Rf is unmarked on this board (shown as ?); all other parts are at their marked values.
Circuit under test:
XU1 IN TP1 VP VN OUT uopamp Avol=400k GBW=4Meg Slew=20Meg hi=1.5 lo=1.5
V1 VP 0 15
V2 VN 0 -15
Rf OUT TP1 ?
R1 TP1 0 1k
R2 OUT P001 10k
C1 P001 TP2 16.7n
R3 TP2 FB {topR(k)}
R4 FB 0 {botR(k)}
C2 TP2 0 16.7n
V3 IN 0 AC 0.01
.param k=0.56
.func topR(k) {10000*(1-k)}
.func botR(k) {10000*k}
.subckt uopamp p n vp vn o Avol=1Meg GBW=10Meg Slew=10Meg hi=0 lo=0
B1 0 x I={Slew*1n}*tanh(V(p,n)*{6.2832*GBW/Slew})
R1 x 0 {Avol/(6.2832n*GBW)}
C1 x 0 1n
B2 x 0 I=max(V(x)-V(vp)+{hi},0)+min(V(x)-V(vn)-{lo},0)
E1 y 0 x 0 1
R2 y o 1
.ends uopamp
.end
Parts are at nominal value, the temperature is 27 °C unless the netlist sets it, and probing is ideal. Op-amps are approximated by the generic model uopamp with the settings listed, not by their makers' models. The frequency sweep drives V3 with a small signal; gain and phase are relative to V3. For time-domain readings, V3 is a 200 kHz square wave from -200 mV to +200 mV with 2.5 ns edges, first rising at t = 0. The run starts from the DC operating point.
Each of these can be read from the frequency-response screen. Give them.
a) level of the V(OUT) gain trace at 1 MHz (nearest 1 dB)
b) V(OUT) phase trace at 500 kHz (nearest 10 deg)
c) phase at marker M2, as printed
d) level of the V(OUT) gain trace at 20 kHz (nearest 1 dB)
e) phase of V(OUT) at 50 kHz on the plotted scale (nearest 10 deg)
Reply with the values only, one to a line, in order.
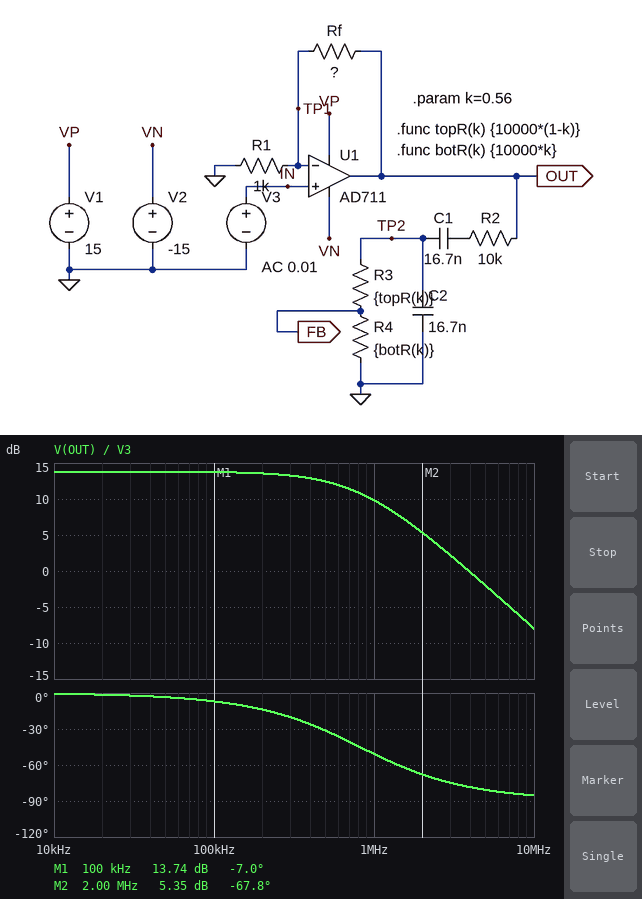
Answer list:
10 dB
-30 deg
-67.8 deg
14 dB
0 deg
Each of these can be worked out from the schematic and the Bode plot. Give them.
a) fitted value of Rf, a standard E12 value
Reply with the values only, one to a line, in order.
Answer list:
3.9 kΩ
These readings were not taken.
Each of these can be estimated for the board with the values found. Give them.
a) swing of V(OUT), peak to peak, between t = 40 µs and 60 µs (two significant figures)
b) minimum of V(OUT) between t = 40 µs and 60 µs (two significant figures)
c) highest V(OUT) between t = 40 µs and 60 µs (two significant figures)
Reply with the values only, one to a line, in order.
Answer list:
2.0 V
-980 mV
980 mV
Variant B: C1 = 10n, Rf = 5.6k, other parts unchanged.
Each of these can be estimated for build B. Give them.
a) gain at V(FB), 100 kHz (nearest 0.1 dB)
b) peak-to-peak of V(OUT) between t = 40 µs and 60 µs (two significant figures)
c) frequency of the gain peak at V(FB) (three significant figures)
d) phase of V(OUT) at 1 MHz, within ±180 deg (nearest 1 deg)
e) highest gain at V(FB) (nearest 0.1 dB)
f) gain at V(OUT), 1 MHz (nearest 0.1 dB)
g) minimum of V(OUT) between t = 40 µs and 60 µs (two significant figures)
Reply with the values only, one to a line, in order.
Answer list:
-29.2 dB
2.6 V
1.23 kHz
-59 deg
0.1 dB
10.7 dB
-1.3 V
